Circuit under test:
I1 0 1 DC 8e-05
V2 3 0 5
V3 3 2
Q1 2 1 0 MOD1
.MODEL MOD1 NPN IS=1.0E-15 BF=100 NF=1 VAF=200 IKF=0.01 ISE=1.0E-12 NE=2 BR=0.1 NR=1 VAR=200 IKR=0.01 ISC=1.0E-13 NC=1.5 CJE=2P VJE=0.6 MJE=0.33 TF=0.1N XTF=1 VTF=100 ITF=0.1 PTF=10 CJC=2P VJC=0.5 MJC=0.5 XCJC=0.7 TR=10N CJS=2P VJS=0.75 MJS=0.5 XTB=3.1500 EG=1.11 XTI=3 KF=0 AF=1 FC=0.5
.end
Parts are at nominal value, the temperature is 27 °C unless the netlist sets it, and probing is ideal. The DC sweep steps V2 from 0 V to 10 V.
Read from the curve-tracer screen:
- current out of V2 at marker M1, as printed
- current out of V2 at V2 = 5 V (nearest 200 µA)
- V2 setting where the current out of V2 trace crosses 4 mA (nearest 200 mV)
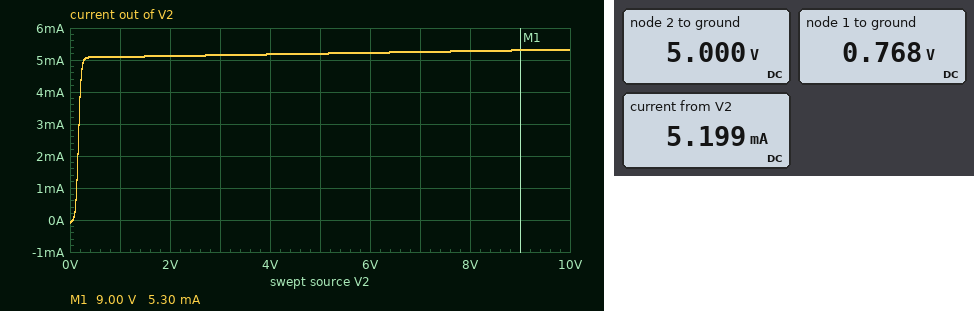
5.30 mA
5.2 mA
200 mV
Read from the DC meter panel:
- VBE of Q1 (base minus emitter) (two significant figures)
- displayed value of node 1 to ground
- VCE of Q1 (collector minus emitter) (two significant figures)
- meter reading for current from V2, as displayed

770 mV
0.768 V
5.0 V
5.199 mA
